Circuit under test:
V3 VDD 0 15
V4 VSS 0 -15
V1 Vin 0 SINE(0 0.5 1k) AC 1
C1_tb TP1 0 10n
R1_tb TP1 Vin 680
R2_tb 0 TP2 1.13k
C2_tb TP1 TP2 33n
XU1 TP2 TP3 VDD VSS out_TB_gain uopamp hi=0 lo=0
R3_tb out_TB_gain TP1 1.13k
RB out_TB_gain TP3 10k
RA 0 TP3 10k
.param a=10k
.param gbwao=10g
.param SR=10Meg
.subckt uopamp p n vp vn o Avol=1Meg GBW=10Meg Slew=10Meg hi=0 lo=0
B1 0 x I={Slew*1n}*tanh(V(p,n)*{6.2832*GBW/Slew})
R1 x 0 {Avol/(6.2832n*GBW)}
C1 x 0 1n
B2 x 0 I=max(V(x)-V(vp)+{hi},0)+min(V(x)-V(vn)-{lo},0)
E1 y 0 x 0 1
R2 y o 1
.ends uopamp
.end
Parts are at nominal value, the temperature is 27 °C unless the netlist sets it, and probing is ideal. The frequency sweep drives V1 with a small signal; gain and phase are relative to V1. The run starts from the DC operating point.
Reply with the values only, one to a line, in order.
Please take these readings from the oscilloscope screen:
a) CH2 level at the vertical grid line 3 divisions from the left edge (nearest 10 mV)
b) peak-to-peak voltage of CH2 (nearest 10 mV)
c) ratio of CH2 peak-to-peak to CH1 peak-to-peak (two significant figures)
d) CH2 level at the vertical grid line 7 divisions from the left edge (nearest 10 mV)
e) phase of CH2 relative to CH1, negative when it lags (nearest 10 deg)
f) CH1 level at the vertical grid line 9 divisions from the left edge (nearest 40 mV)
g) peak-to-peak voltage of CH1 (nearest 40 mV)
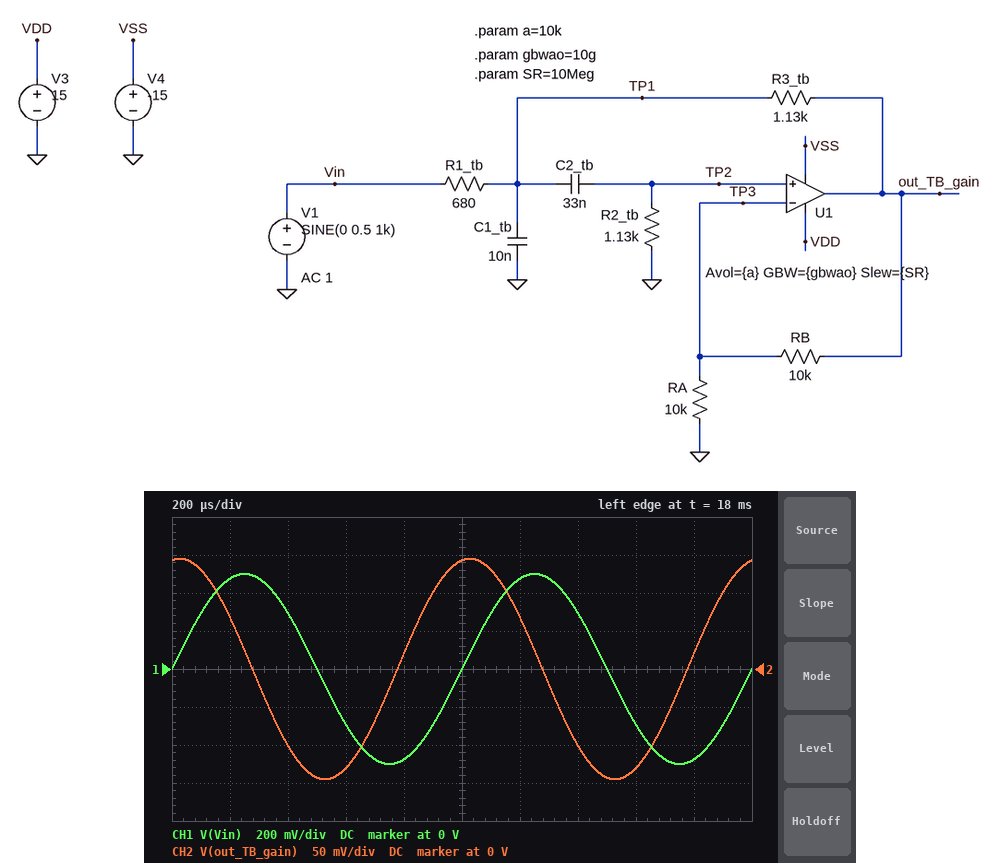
-130 mV
290 mV
0.29
-100 mV
80 deg
-480 mV
1.00 V
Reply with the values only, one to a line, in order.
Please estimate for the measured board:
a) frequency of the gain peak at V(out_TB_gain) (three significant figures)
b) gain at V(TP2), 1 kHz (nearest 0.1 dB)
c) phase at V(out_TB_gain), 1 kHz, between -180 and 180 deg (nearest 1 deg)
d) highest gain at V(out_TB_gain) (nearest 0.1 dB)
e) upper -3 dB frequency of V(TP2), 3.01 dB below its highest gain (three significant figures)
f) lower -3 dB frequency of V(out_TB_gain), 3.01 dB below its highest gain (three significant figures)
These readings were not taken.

12.6 kHz
-16.8 dB
80 deg
4.6 dB
32.4 kHz
4.91 kHz
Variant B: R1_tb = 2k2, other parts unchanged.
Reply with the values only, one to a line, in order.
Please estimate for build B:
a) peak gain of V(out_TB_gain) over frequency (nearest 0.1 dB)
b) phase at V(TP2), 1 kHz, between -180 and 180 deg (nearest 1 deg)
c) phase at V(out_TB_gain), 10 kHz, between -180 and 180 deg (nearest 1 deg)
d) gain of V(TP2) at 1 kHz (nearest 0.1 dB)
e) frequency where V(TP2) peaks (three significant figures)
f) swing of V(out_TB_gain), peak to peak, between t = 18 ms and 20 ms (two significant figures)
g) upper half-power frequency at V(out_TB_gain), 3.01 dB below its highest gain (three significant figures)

2.0 dB
83 deg
-5 deg
-22.0 dB
9.51 kHz
160 mV
16.8 kHz
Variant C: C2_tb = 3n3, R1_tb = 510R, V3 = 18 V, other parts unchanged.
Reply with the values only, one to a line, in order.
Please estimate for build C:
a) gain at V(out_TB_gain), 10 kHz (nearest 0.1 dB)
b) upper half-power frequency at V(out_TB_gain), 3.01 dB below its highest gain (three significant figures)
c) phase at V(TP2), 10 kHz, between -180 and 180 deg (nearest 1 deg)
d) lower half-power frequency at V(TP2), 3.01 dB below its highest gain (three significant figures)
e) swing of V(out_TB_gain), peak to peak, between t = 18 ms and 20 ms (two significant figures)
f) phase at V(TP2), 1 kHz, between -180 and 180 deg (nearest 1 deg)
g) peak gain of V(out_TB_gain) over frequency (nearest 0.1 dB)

-10.0 dB
93.9 kHz
68 deg
20.5 kHz
32 mV
88 deg
-1.5 dB
